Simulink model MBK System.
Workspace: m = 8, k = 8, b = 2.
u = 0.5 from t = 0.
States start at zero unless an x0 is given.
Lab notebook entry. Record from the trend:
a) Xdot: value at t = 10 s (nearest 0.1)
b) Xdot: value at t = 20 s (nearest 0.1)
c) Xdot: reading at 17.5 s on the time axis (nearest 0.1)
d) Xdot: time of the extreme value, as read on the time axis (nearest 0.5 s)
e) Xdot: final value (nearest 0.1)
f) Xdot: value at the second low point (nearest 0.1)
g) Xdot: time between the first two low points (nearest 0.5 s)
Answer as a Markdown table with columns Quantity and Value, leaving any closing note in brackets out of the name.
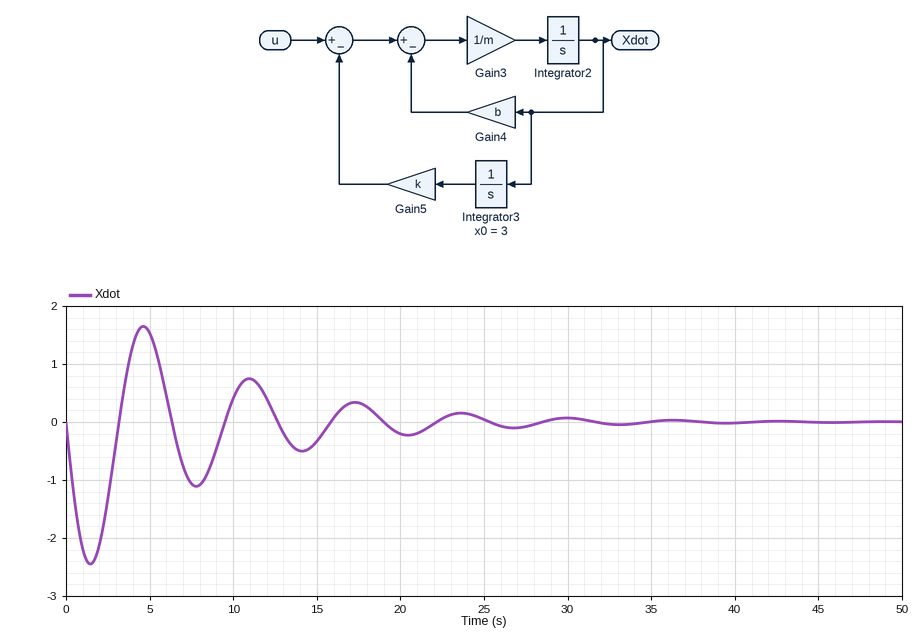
| Quantity | Value |
|---|---|
| Xdot: value at t = 10 s | 0.4 |
| Xdot: value at t = 20 s | -0.2 |
| Xdot: reading at 17.5 s on the time axis | 0.3 |
| Xdot: time of the extreme value, as read on the time axis | 1.5 s |
| Xdot: final value | 0.0 |
| Xdot: value at the second low point | -1.1 |
| Xdot: time between the first two low points | 6.5 s |
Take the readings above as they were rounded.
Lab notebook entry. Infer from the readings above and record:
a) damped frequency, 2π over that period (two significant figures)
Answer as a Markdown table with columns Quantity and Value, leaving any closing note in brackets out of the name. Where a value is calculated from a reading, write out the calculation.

| Quantity | Value |
|---|---|
| damped frequency, 2π over that period | 2π / 6.5 = 0.97 rad/s |
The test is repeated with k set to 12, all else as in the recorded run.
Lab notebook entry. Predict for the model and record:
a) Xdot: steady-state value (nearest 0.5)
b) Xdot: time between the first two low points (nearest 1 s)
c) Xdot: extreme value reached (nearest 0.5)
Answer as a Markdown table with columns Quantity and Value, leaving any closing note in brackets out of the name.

| Quantity | Value |
|---|---|
| Xdot: steady-state value | 0.0 |
| Xdot: time between the first two low points | 5 s |
| Xdot: extreme value reached | -3.0 |
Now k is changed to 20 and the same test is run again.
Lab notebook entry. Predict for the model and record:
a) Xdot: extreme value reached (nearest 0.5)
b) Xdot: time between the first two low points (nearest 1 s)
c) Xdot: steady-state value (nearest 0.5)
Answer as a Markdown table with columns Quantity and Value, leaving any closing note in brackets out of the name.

| Quantity | Value |
|---|---|
| Xdot: extreme value reached | -4.0 |
| Xdot: time between the first two low points | 4 s |
| Xdot: steady-state value | 0.0 |
